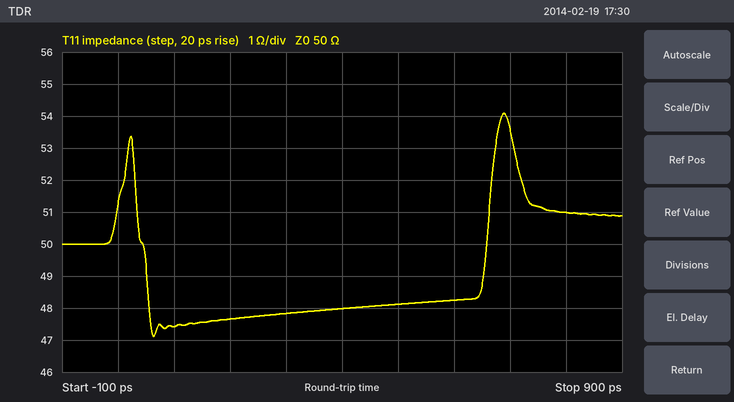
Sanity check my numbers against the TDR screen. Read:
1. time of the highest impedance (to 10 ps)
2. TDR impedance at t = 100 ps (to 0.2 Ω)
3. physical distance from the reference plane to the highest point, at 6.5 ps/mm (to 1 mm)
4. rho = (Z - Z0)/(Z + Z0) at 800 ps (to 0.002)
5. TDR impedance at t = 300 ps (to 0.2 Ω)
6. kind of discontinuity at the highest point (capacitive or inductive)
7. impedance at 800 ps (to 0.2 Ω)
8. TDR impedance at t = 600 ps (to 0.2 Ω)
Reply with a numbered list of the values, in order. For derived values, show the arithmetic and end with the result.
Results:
1. 690 ps
2. 47.4 Ω
3. 690 ps / 2 / 6.5 ps/mm ≈ 53 mm
4. (51 − 50)/(51 + 50) ≈ +0.010
5. 47.8 Ω
6. inductive
7. 51.0 Ω
8. 48.2 Ω
